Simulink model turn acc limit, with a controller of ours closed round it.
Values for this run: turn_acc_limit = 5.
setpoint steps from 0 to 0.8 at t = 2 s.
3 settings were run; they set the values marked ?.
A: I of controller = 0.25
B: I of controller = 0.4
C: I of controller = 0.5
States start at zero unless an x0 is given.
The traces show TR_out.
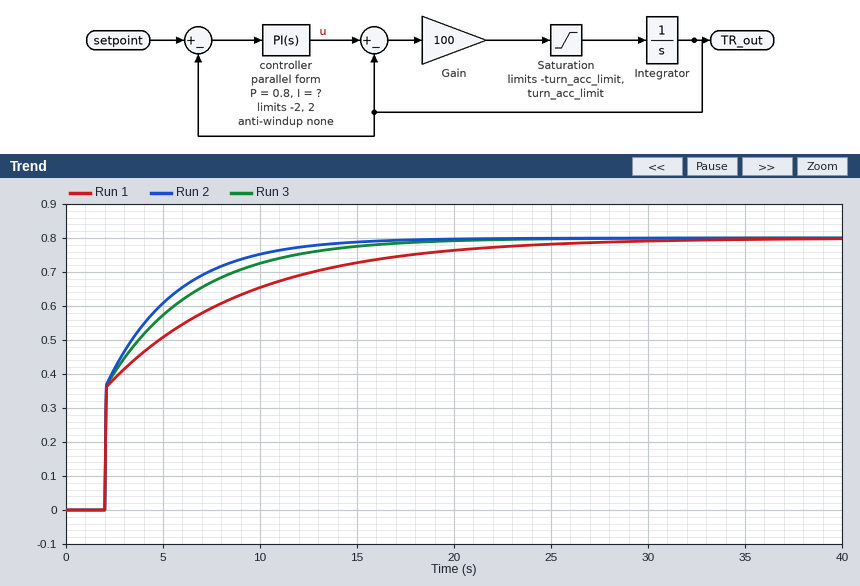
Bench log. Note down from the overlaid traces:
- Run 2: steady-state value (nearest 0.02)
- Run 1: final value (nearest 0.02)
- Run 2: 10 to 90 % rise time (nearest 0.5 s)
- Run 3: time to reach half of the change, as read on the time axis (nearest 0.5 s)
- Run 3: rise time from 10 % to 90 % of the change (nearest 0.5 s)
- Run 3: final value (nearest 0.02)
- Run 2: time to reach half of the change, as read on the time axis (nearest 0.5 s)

0.80
0.80
6.0 s
2.5 s
7.5 s
0.80
2.5 s
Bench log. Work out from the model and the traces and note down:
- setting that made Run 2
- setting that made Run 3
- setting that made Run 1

C
B
A
